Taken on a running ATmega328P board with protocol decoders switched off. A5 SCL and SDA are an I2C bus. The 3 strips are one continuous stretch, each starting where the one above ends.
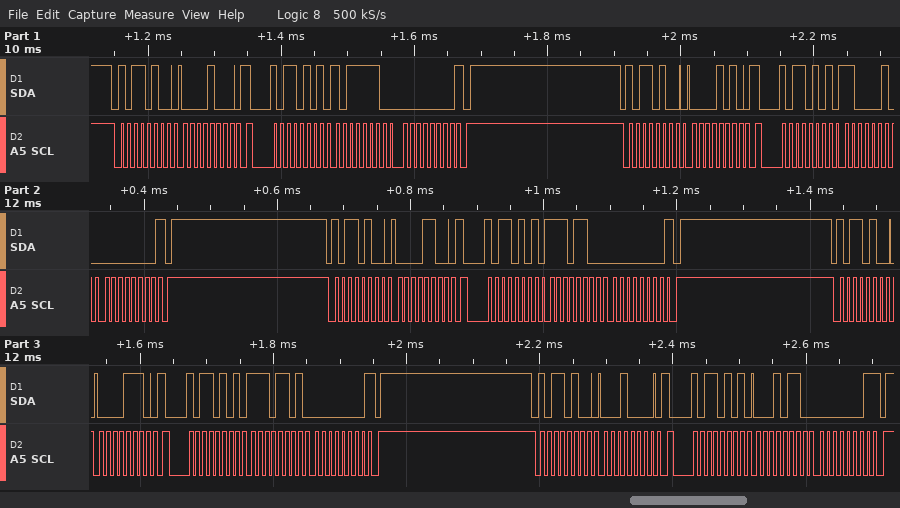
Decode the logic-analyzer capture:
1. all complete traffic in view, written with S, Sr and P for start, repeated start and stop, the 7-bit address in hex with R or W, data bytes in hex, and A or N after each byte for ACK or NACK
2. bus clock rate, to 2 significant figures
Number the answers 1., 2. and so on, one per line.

1. S 5AW A 08 A Sr 5AR A BE A 00 N P S 5AW A 0A A Sr 5AR A C2 A 00 N P S 5AW A 0C A Sr 5AR A EC A 00 N P S 5AW A 0E A Sr 5AR A ED A 00 N P S 5AW A 10 A Sr 5AR A 16 A 01 N P
2. 100 kHz
